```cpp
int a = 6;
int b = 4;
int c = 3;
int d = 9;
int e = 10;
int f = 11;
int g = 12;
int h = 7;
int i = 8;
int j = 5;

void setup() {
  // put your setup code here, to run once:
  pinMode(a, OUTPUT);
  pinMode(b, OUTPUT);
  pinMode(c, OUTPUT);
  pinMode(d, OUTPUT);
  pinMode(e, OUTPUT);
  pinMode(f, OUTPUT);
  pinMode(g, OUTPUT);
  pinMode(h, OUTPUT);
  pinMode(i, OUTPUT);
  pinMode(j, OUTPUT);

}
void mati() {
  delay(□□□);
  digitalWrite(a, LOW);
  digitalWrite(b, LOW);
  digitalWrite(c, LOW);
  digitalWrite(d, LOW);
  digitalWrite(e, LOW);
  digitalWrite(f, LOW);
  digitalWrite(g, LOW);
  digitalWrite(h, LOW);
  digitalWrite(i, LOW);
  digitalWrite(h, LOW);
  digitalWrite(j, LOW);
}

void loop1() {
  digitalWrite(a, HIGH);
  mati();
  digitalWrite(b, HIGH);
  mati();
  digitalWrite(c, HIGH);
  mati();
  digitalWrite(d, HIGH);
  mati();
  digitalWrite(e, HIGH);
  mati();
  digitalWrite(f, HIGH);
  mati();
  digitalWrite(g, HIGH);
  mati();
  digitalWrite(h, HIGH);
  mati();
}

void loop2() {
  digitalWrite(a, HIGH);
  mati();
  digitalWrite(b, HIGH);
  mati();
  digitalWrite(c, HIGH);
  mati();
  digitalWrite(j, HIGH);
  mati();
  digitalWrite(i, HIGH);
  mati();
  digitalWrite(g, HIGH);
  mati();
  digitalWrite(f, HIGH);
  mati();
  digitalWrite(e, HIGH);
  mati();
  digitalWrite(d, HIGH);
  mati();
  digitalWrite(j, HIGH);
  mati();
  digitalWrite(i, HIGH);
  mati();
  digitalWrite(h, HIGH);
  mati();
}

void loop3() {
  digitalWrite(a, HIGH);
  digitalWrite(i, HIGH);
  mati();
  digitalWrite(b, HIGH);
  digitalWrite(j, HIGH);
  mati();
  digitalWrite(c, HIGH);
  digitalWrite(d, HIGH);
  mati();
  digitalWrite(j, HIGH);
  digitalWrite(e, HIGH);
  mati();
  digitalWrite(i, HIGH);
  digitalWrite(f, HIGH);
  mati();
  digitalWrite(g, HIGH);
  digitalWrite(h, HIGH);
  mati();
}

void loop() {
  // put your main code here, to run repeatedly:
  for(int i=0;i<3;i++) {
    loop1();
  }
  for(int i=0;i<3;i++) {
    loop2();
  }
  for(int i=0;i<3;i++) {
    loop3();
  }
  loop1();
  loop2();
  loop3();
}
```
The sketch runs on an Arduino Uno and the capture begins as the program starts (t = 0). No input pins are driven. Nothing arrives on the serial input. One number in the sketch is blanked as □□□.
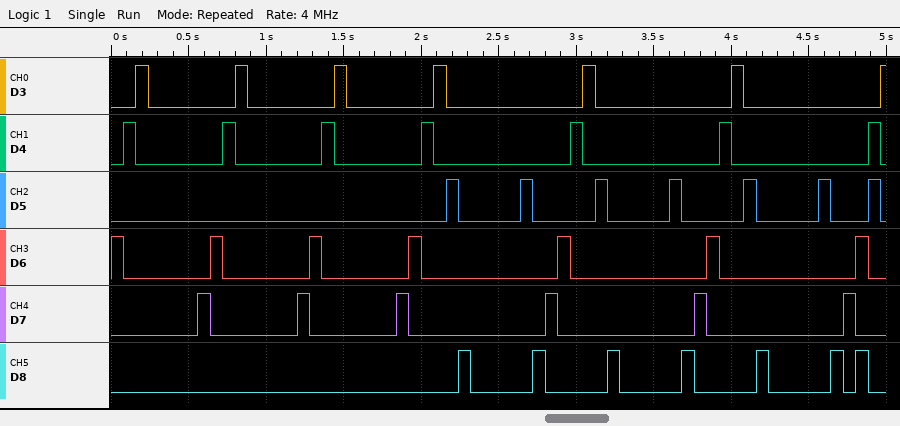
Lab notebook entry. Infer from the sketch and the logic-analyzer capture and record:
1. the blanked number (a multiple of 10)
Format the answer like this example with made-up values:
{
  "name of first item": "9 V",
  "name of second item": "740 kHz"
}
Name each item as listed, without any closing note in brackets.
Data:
{
  "the blanked number": "80"
}
